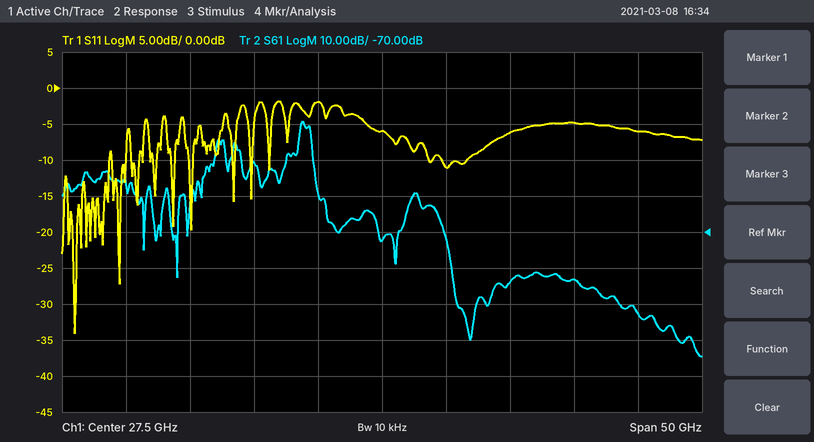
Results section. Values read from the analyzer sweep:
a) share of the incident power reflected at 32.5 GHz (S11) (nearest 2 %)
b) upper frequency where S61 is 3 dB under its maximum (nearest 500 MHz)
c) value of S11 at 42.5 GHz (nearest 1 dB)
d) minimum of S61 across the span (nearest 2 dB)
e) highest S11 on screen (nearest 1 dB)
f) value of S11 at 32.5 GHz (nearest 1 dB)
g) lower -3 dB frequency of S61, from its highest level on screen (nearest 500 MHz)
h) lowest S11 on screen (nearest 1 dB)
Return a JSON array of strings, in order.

["8 %", "22.0 GHz", "-5 dB", "-104 dB", "-2 dB", "-11 dB", "21.0 GHz", "-34 dB"]
